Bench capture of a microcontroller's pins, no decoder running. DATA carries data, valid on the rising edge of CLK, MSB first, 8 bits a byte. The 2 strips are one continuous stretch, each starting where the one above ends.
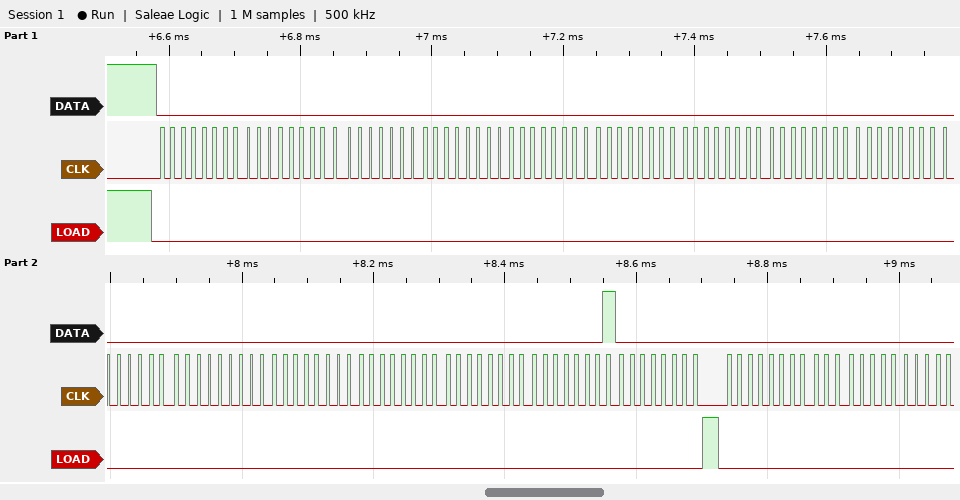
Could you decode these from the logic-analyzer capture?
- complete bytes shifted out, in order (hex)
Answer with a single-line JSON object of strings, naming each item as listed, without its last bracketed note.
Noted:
{"complete bytes shifted out, in order": "00 00 00 00 00 00 00 00 00 00 00 00 00 00 01 00 00 00"}
